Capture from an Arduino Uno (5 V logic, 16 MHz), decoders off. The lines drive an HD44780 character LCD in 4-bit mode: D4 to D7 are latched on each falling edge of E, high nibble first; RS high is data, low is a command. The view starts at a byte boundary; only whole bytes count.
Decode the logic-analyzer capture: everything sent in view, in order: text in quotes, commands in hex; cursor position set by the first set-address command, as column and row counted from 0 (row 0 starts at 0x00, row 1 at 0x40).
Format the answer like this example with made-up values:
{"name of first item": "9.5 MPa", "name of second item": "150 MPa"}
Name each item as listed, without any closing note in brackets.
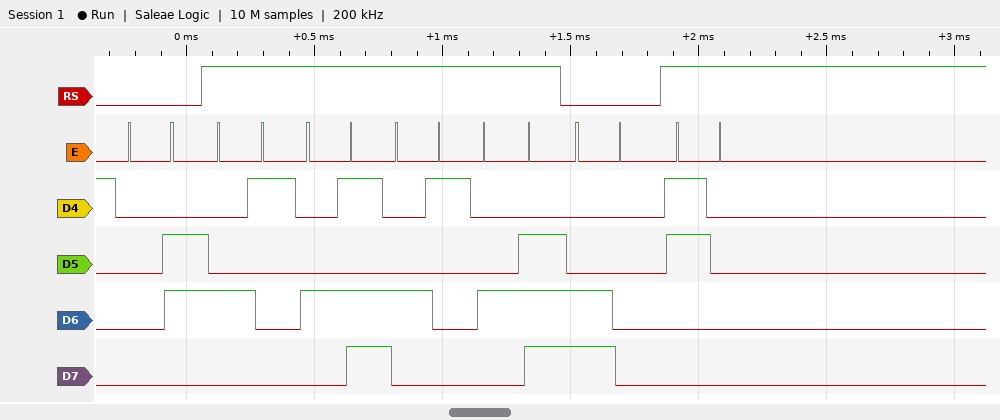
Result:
{"everything sent in view, in order: text in quotes, commands in hex": "0x06 \"AMAN\" 0xC0 \"0\"", "cursor position set by the first set-address command, as column and row counted from 0": "column 0, row 1"}
